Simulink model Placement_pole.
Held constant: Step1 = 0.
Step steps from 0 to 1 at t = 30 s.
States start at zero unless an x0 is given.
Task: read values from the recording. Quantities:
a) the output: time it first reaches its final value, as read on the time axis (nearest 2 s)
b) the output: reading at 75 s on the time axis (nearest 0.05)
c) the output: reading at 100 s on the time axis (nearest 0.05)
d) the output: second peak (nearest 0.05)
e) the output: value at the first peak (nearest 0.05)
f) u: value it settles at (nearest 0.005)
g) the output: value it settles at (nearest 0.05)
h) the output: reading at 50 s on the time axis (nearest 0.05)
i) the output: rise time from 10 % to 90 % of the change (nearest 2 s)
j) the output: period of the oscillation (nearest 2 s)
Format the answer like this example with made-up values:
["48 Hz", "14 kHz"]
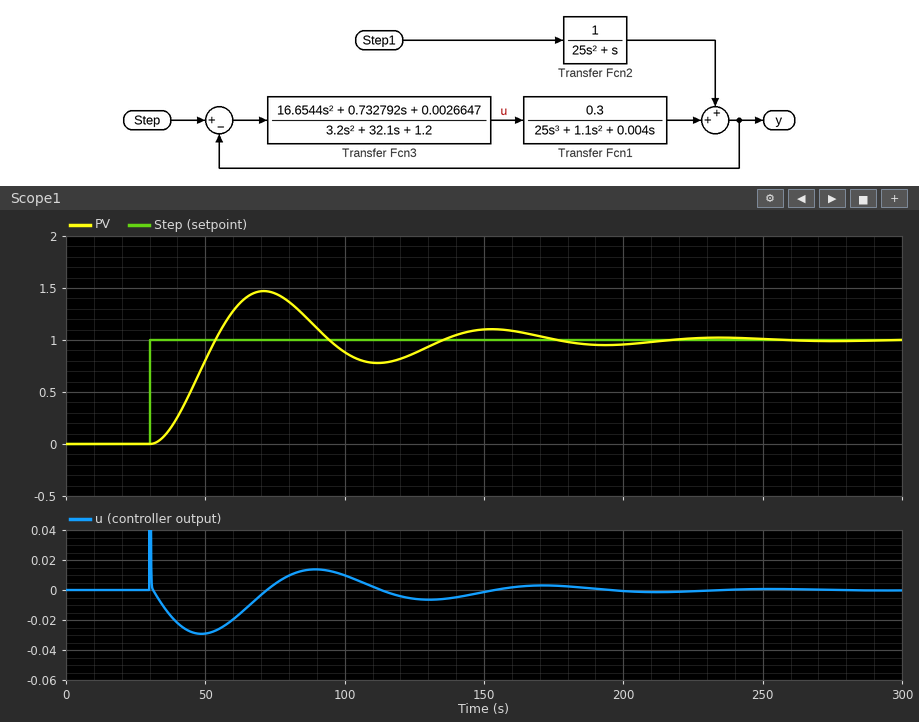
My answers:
["54 s", "1.45", "0.90", "1.10", "1.45", "0.000", "1.00", "0.80", "16 s", "82 s"]
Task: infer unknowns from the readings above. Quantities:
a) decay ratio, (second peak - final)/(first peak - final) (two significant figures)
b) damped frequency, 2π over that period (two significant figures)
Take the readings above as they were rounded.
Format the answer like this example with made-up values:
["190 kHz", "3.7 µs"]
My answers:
["0.22", "0.077 rad/s"]
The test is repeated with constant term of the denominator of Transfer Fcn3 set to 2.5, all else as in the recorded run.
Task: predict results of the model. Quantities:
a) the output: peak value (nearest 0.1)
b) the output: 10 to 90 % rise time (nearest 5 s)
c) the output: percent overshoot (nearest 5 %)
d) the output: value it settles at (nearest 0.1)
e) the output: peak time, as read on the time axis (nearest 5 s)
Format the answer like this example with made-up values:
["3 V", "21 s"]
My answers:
["1.2", "20 s", "15 %", "1.0", "75 s"]
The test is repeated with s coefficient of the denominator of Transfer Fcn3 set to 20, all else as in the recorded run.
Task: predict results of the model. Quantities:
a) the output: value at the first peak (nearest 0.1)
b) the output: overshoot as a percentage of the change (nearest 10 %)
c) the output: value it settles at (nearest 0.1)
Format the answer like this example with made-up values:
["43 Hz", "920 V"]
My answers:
["1.4", "40 %", "1.0"]
